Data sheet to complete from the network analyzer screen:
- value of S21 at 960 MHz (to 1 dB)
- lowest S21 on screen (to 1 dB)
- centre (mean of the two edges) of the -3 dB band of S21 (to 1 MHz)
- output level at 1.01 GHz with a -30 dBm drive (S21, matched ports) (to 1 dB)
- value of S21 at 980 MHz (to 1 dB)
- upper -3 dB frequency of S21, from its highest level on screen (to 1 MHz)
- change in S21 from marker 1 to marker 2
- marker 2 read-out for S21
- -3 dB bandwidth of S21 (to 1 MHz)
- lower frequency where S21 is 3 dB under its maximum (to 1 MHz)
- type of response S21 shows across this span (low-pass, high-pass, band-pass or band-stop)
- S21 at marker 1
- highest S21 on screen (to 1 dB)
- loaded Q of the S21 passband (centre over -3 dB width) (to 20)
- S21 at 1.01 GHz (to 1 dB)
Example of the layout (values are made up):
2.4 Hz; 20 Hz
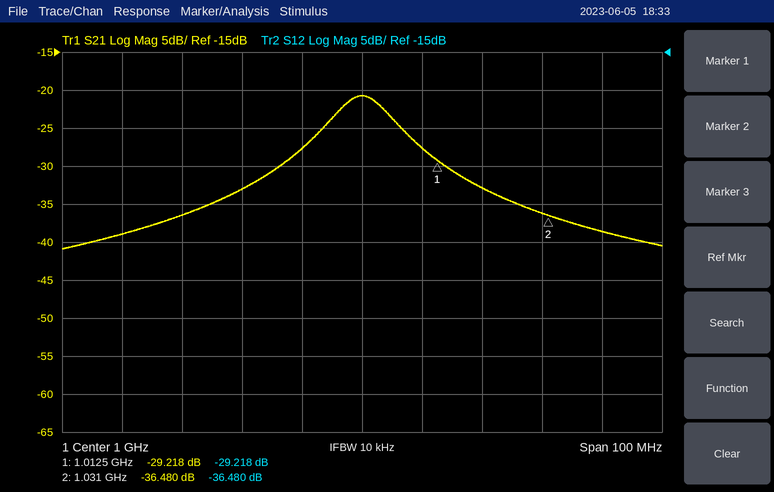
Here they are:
-39 dB; -41 dB; 1.000 GHz; -58 dBm; -33 dB; 1.005 GHz; -7.262 dB; -36.480 dB; 10 MHz; 995 MHz; band-pass; -29.218 dB; -21 dB; 100; -28 dB
